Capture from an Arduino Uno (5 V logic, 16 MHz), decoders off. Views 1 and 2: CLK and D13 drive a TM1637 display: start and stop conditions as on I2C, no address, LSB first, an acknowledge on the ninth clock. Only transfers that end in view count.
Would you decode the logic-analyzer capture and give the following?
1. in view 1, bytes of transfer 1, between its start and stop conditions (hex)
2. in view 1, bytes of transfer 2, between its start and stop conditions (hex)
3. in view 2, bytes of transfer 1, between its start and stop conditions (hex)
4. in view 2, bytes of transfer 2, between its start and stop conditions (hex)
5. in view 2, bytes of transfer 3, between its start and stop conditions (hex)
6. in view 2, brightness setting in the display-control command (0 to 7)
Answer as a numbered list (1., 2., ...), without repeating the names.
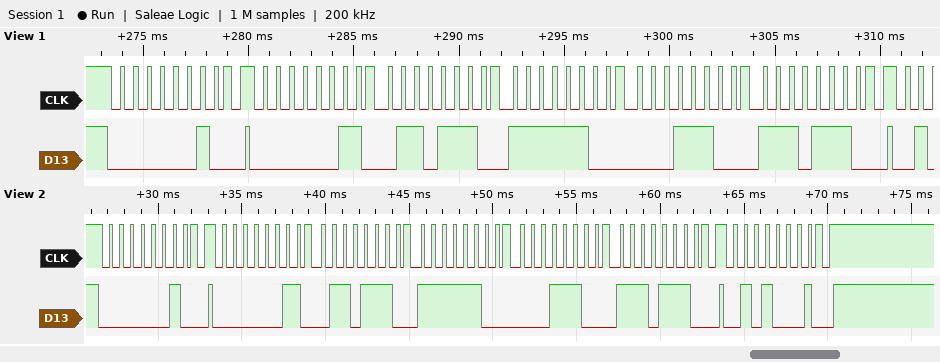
1. 40
2. C0 76 3F 38 77
3. 40
4. C0 76 3F 38 77
5. 8A
6. 2
